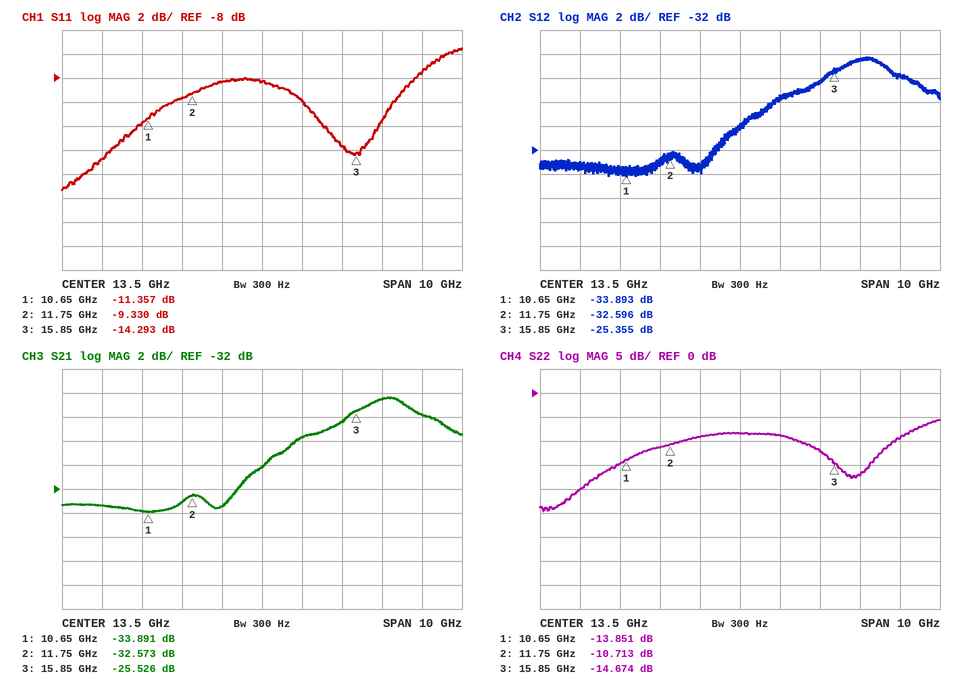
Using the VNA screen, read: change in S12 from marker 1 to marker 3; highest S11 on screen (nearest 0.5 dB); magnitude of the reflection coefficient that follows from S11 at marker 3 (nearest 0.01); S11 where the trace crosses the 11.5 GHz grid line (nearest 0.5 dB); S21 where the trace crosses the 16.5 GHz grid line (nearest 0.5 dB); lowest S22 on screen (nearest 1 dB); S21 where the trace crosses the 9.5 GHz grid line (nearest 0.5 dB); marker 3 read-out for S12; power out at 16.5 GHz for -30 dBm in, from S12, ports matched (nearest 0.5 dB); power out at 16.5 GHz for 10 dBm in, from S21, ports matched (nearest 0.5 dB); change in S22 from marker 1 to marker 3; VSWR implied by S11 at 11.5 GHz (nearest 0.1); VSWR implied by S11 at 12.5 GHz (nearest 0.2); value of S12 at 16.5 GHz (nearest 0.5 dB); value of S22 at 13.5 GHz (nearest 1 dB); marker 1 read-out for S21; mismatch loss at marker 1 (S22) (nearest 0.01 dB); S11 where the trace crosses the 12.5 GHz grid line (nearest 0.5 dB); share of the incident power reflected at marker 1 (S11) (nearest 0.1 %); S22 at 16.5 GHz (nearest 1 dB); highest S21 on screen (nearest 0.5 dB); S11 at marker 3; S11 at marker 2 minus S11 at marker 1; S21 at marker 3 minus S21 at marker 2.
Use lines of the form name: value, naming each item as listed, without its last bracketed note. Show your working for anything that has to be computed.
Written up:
change in S12 from marker 1 to marker 3: -25.355 − (-33.893) = 8.538 dB
highest S11 on screen: -5.5 dB
magnitude of the reflection coefficient that follows from S11 at marker 3: 10^(-14.293/20) ≈ 0.19
S11 where the trace crosses the 11.5 GHz grid line: -9.5 dB
S21 where the trace crosses the 16.5 GHz grid line: -24.5 dB
lowest S22 on screen: -25 dB
S21 where the trace crosses the 9.5 GHz grid line: -33.5 dB
marker 3 read-out for S12: -25.355 dB
power out at 16.5 GHz for -30 dBm in, from S12, ports matched: -30 dBm + (-24.5 dB) = -54.5 dBm
power out at 16.5 GHz for 10 dBm in, from S21, ports matched: 10 dBm + (-24.5 dB) = -14.5 dBm
change in S22 from marker 1 to marker 3: -14.674 − (-13.851) = -0.823 dB
VSWR implied by S11 at 11.5 GHz: |Γ| = 10^(-9.5/20) = 0.3350; VSWR = (1 + 0.3350)/(1 − 0.3350) ≈ 2.0
VSWR implied by S11 at 12.5 GHz: |Γ| = 10^(-8.5/20) = 0.3758; VSWR = (1 + 0.3758)/(1 − 0.3758) ≈ 2.2
value of S12 at 16.5 GHz: -24.5 dB
value of S22 at 13.5 GHz: -8 dB
marker 1 read-out for S21: -33.891 dB
mismatch loss at marker 1 (S22): −10 log10(1 − 10^(-13.851/10)) ≈ 0.18 dB
S11 where the trace crosses the 12.5 GHz grid line: -8.5 dB
share of the incident power reflected at marker 1 (S11): 10^(-11.357/10) ≈ 7.3 %
S22 at 16.5 GHz: -17 dB
highest S21 on screen: -24.5 dB
S11 at marker 3: -14.293 dB
S11 at marker 2 minus S11 at marker 1: -9.33 − (-11.357) = 2.027 dB
S21 at marker 3 minus S21 at marker 2: -25.526 − (-32.573) = 7.047 dB
